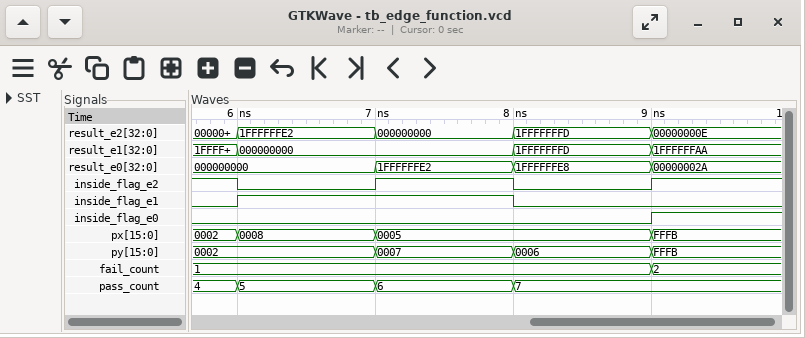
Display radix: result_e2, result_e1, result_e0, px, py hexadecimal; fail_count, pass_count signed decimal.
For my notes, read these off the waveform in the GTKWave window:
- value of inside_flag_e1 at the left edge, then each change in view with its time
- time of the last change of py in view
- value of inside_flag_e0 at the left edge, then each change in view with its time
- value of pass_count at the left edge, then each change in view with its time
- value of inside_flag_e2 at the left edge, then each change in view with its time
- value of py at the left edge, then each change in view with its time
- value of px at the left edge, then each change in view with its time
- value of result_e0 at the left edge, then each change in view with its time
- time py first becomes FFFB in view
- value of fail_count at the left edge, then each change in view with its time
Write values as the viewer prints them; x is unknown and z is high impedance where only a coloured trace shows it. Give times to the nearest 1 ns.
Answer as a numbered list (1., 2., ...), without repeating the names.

1. 0, 1 at 6 ns, 0 at 8 ns
2. 9 ns
3. 0, 1 at 9 ns
4. 4, 5 at 6 ns, 6 at 7 ns, 7 at 8 ns
5. 1, 0 at 6 ns, 1 at 7 ns, 0 at 8 ns, 1 at 9 ns
6. 0002, 0007 at 7 ns, 0006 at 8 ns, FFFB at 9 ns
7. 0002, 0008 at 6 ns, 0005 at 7 ns, FFFB at 9 ns
8. 000000000, 1FFFFFFE2 at 7 ns, 1FFFFFFE8 at 8 ns, 00000002A at 9 ns
9. 9 ns
10. 1, 2 at 9 ns
